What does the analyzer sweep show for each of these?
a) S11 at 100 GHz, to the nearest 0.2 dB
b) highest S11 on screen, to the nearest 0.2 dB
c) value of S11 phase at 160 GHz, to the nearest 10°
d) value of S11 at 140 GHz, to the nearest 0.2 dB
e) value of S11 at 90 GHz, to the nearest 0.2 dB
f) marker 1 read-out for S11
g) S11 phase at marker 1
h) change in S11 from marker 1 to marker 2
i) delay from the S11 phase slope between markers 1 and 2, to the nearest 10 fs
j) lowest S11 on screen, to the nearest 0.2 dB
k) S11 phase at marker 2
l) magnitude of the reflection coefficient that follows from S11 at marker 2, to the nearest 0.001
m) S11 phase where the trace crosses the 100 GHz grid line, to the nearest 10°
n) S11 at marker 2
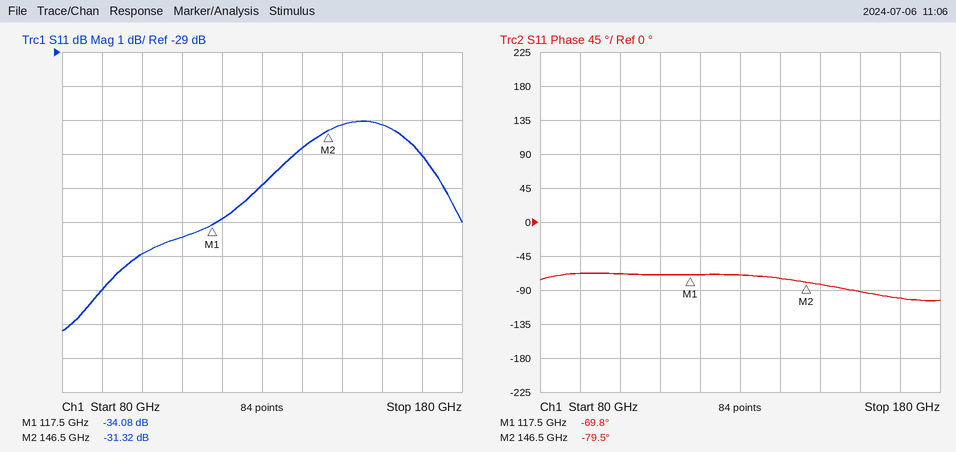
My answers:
-35.0 dB
-31.0 dB
-90°
-31.8 dB
-36.0 dB
-34.08 dB
-69.8°
2.76 dB
930 fs
-37.2 dB
-79.5°
0.027
-70°
-31.32 dB
